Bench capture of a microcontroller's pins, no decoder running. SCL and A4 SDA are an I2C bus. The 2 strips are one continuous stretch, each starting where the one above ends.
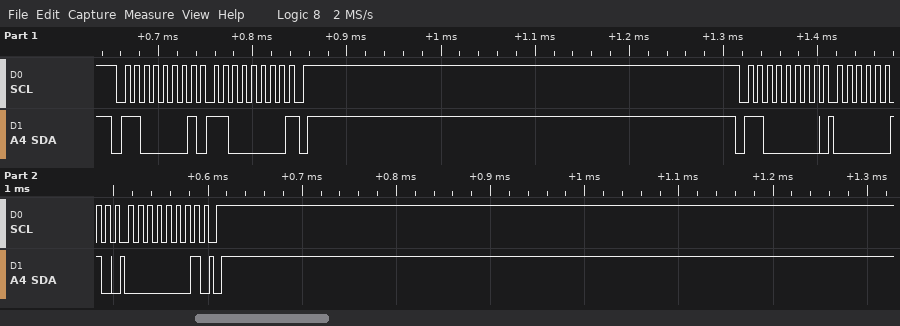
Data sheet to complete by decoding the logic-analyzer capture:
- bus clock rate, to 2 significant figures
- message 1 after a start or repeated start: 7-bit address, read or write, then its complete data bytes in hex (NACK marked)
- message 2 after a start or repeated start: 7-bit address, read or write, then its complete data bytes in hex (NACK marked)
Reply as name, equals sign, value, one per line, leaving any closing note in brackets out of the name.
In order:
bus clock rate, to 2 significant figures = 100 kHz
message 1 after a start or repeated start: 7-bit address, read or write, then its complete data bytes in hex = 0x60 read: C0 NACK
message 2 after a start or repeated start: 7-bit address, read or write, then its complete data bytes in hex = 0x60 write: 02 01
